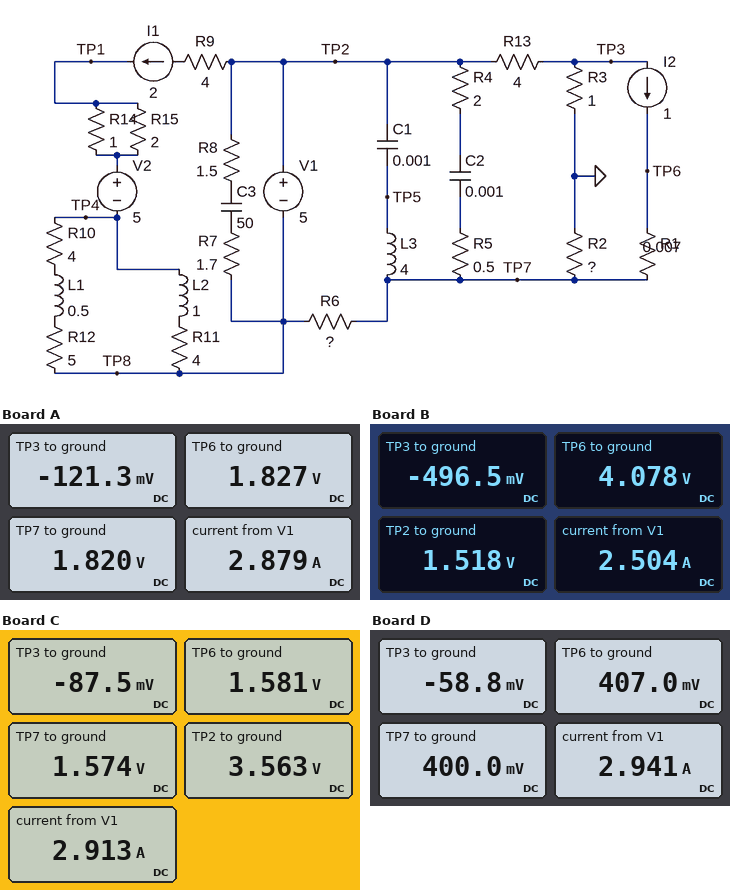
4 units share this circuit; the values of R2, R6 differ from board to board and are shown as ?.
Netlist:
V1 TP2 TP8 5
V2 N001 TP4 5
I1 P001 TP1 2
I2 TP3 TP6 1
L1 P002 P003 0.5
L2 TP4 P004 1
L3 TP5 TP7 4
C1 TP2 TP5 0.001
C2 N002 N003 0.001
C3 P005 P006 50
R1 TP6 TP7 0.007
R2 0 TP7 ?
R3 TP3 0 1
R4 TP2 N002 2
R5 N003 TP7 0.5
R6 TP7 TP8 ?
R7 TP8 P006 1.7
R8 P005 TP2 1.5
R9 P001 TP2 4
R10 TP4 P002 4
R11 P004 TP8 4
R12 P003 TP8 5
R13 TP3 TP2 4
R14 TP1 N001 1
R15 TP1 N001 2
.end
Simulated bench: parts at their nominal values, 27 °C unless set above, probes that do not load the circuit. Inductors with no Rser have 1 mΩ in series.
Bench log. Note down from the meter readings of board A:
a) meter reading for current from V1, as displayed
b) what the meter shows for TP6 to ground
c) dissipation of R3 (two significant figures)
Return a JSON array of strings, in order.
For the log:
["2.879 A", "1.827 V", "15 mW"]
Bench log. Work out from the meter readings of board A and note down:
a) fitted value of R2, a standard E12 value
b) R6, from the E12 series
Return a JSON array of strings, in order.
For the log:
["15 Ω", "3.9 Ω"]
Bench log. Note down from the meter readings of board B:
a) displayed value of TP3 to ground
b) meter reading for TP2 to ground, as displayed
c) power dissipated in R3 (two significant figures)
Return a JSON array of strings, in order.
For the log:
["-496.5 mV", "1.518 V", "250 mW"]
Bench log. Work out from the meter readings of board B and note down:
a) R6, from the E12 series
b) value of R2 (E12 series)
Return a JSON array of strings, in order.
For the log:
["15 Ω", "8.2 Ω"]
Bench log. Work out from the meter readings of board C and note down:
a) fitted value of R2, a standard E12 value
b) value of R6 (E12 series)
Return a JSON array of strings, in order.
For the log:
["18 Ω", "3.3 Ω"]
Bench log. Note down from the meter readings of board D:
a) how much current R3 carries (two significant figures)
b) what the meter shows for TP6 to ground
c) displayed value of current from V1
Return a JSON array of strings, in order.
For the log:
["59 mA", "407.0 mV", "2.941 A"]
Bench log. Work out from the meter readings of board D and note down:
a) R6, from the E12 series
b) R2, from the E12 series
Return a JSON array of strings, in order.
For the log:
["1.8 Ω", "6.8 Ω"]
